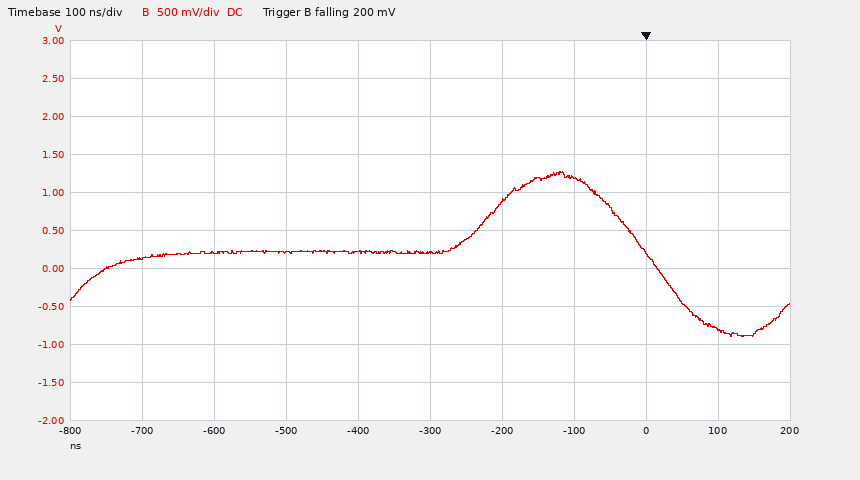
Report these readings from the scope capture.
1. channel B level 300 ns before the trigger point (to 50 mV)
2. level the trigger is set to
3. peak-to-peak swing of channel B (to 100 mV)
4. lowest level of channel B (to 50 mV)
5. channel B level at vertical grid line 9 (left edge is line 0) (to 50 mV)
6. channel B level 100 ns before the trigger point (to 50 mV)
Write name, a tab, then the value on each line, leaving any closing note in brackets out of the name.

channel B level 300 ns before the trigger point	200 mV
level the trigger is set to	200 mV
peak-to-peak swing of channel B	2.20 V
lowest level of channel B	-900 mV
channel B level at vertical grid line 9 (left edge is line 0)	-800 mV
channel B level 100 ns before the trigger point	1.20 V
